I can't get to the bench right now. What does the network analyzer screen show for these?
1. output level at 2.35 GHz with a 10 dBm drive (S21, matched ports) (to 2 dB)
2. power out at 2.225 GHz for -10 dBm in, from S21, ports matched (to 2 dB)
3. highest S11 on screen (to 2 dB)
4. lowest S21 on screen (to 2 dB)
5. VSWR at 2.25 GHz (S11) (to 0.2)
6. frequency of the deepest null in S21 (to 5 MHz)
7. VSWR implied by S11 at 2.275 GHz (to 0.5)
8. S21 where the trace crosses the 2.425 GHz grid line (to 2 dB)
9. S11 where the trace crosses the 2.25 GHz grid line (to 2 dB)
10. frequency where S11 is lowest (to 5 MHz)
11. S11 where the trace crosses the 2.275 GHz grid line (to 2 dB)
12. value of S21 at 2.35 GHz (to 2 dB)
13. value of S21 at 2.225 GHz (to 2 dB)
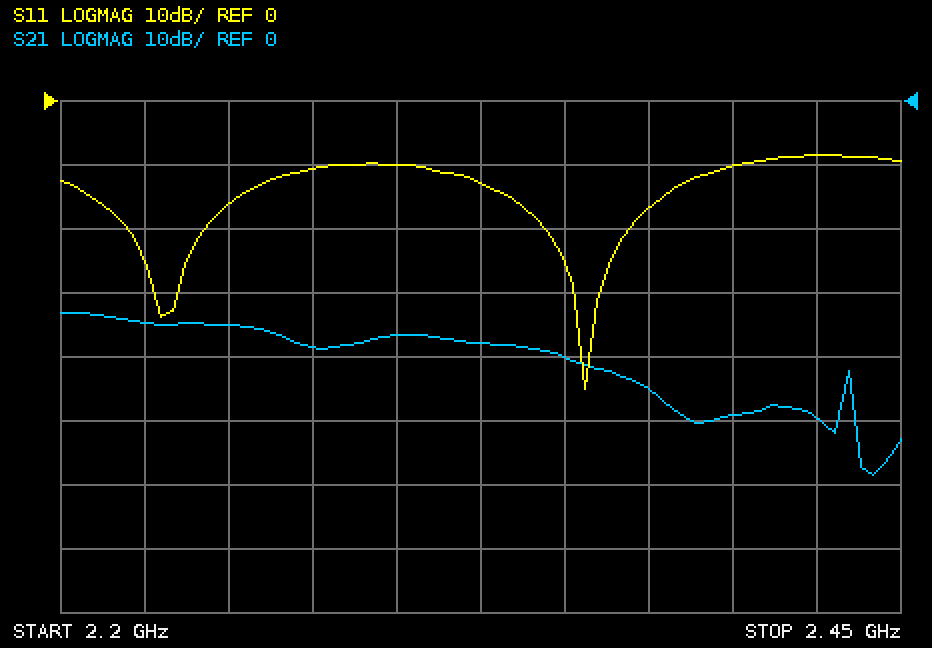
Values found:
-30 dBm
-44 dBm
-8 dB
-58 dB
1.4
2.440 GHz
2.0
-50 dB
-16 dB
2.355 GHz
-10 dB
-40 dB
-34 dB
